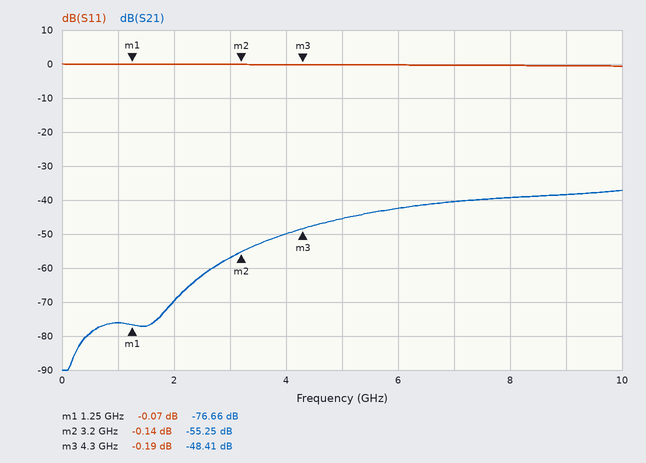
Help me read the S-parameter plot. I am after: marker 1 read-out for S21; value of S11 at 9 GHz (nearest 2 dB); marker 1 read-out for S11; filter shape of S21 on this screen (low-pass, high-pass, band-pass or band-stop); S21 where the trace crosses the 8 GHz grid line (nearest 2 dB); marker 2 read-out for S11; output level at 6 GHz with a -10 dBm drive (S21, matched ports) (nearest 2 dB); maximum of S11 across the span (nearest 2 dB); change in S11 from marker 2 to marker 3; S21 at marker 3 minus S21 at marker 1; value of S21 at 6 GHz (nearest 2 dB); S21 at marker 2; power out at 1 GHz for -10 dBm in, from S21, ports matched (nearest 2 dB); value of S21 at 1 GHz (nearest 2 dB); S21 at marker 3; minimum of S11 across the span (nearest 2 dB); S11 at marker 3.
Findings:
-76.66 dB
0 dB
-0.07 dB
high-pass
-40 dB
-0.14 dB
-52 dBm
0 dB
-0.05 dB
28.25 dB
-42 dB
-55.25 dB
-86 dBm
-76 dB
-48.41 dB
0 dB
-0.19 dB
